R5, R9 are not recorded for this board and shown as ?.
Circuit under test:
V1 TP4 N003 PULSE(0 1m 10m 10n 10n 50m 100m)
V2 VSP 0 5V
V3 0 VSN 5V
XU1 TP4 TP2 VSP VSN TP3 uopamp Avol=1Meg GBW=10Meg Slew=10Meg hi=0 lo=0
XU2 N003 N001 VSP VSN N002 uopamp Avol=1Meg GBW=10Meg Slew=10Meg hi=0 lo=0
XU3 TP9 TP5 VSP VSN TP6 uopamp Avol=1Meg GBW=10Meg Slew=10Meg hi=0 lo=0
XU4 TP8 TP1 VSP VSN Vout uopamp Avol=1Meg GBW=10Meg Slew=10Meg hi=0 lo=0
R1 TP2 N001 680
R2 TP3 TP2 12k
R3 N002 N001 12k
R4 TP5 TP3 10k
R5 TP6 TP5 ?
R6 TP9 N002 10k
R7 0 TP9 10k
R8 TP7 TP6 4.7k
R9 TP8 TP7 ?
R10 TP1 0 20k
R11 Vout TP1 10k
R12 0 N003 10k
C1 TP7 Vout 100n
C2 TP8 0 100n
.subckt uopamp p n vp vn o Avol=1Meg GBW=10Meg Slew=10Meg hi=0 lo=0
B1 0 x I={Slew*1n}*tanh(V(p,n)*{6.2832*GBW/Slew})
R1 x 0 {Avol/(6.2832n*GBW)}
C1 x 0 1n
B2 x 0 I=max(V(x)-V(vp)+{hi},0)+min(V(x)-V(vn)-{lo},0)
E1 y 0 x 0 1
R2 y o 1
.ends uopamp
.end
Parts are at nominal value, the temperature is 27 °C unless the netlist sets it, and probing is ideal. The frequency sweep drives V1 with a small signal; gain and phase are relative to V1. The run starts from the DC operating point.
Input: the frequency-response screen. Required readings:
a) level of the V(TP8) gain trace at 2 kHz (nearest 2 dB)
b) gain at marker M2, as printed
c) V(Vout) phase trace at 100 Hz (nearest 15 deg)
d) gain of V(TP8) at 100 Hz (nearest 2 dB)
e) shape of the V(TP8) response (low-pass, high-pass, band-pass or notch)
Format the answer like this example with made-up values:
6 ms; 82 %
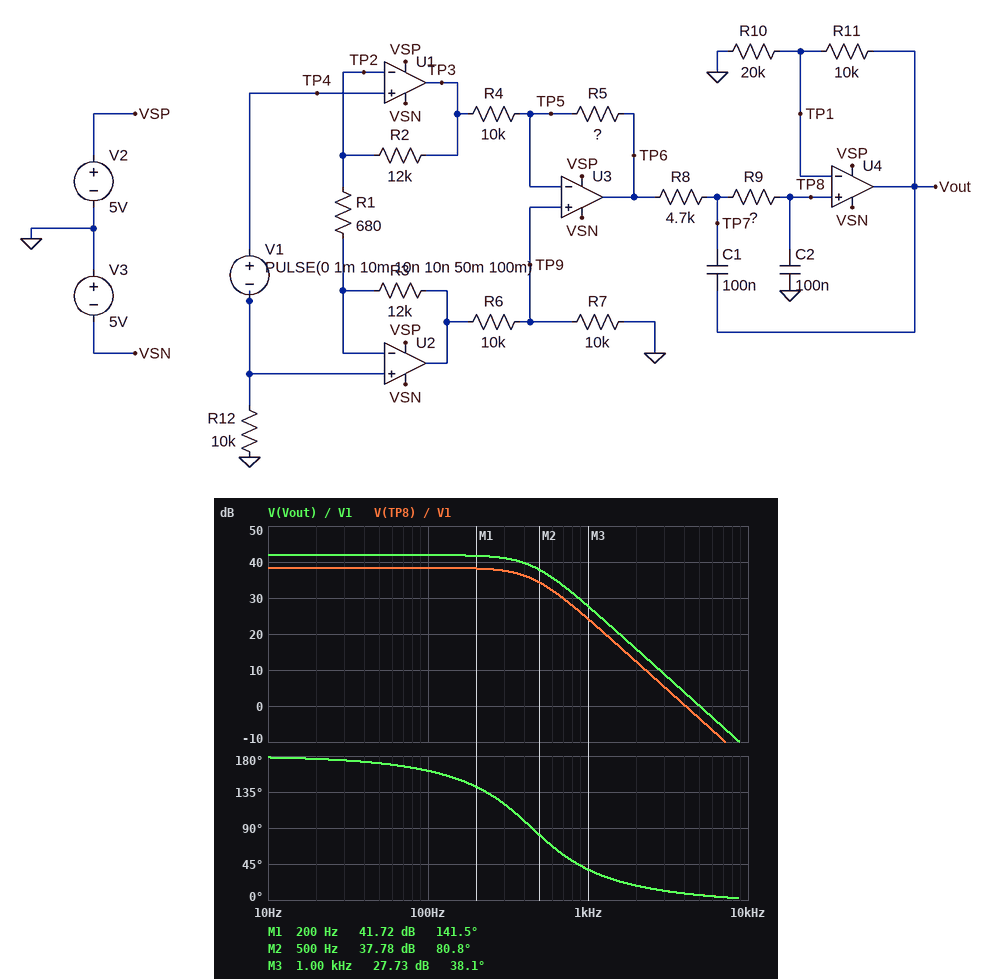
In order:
12 dB; 37.78 dB; 165 deg; 38 dB; low-pass
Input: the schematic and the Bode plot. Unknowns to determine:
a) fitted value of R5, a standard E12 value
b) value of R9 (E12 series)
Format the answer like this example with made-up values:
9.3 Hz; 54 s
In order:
27 kΩ; 2.7 kΩ
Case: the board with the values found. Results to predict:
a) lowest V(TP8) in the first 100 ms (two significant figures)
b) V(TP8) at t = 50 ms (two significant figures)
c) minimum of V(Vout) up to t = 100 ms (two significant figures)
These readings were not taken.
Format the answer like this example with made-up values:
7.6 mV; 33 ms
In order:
-87 mV; -83 mV; -130 mV
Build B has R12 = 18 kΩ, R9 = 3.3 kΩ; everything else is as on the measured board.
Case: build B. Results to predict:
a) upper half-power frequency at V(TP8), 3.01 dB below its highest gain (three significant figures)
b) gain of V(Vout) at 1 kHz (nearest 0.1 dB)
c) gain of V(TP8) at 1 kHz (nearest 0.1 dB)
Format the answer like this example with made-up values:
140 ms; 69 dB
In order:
398 Hz; 26.0 dB; 22.5 dB
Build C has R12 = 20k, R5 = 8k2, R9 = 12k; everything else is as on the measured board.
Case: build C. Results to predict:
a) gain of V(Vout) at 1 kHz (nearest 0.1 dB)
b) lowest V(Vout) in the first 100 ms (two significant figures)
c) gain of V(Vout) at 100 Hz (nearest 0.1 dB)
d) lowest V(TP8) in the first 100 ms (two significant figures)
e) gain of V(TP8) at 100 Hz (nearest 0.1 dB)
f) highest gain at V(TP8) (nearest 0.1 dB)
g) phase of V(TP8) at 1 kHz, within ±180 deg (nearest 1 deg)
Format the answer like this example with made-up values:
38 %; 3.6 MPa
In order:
6.2 dB; -47 mV; 31.9 dB; -31 mV; 28.4 dB; 29.9 dB; 23 deg
